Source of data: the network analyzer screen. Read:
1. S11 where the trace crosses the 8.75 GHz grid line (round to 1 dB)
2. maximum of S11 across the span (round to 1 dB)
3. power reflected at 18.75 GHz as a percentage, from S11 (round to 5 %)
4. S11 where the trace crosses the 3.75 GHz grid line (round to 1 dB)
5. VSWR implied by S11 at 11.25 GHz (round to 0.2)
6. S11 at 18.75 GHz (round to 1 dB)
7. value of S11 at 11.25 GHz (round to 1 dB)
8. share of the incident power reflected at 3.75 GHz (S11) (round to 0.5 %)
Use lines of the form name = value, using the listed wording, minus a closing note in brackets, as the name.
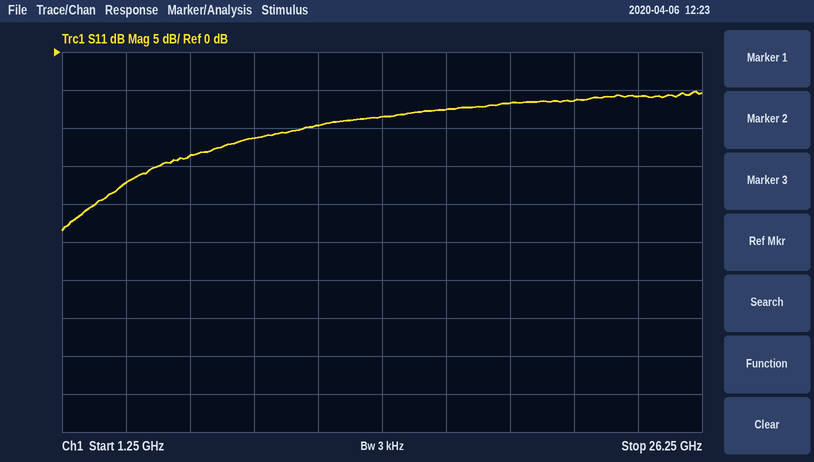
S11 where the trace crosses the 8.75 GHz grid line = -11 dB
maximum of S11 across the span = -5 dB
power reflected at 18.75 GHz as a percentage, from S11 = 20 %
S11 where the trace crosses the 3.75 GHz grid line = -17 dB
VSWR implied by S11 at 11.25 GHz = 2.0
S11 at 18.75 GHz = -7 dB
value of S11 at 11.25 GHz = -10 dB
share of the incident power reflected at 3.75 GHz (S11) = 2.0 %
